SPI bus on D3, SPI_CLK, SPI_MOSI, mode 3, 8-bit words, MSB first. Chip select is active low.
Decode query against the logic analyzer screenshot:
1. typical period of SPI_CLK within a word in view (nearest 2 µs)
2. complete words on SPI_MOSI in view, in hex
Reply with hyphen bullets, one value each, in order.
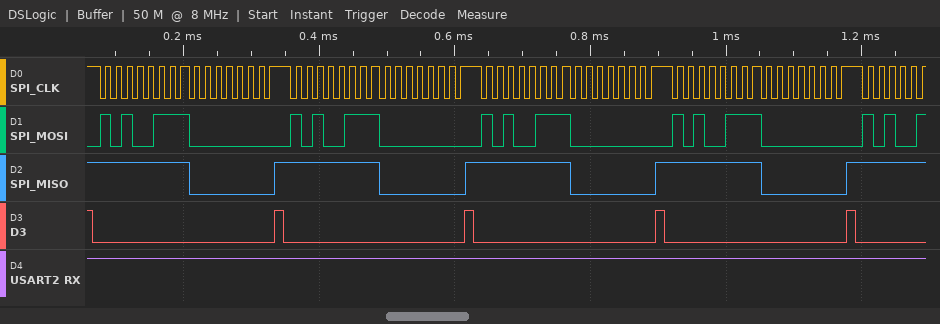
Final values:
- 16 µs
- A7, 00, A7, 00, A7, 00, A7, 00
